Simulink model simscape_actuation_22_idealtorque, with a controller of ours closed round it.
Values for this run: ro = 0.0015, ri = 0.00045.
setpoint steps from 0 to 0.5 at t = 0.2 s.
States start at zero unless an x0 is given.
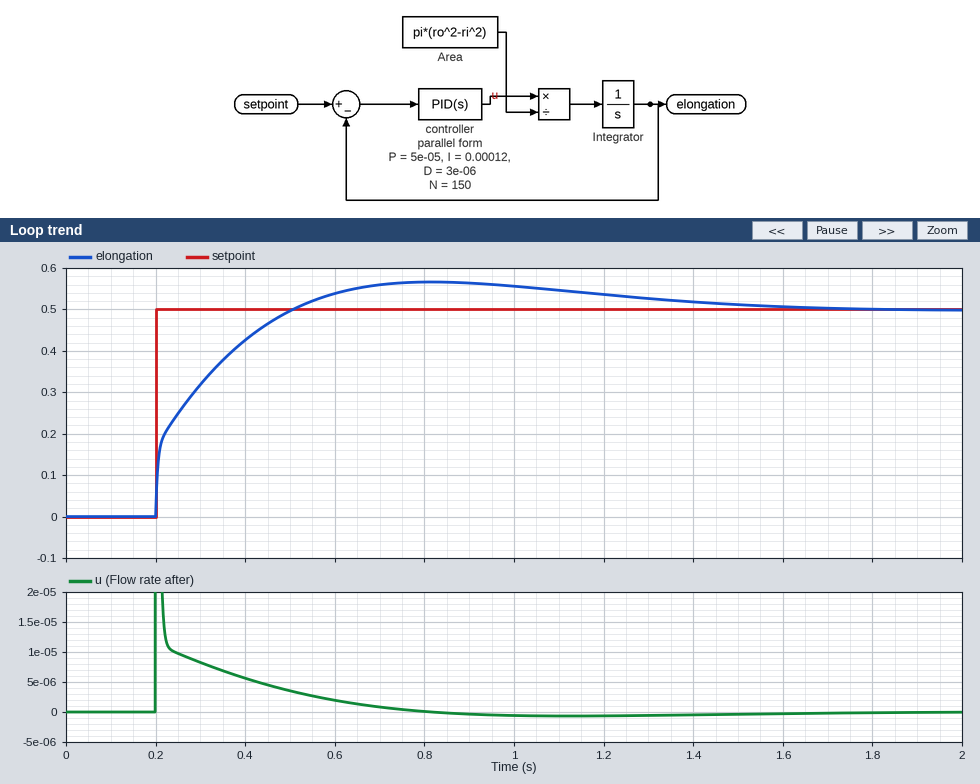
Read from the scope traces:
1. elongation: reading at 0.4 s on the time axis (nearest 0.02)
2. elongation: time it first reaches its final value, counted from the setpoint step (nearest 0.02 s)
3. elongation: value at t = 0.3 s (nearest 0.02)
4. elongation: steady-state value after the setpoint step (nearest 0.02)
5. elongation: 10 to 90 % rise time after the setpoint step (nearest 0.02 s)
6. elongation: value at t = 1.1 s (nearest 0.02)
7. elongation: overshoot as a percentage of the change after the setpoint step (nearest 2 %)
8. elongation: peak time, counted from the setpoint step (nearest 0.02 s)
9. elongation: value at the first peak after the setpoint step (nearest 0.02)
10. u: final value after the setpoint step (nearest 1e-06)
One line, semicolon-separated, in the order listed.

0.42; 0.30 s; 0.32; 0.50; 0.22 s; 0.54; 14 %; 0.62 s; 0.56; 0.000000
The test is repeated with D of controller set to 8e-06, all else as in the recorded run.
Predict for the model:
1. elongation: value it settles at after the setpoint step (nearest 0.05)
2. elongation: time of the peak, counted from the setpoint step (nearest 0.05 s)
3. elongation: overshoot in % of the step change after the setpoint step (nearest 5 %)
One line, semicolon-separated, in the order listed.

0.50; 0.80 s; 10 %
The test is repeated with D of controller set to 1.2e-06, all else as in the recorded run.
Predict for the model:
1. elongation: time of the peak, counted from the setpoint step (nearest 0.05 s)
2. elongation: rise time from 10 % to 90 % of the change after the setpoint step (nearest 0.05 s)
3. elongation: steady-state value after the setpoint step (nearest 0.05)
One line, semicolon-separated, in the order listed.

0.55 s; 0.20 s; 0.50
